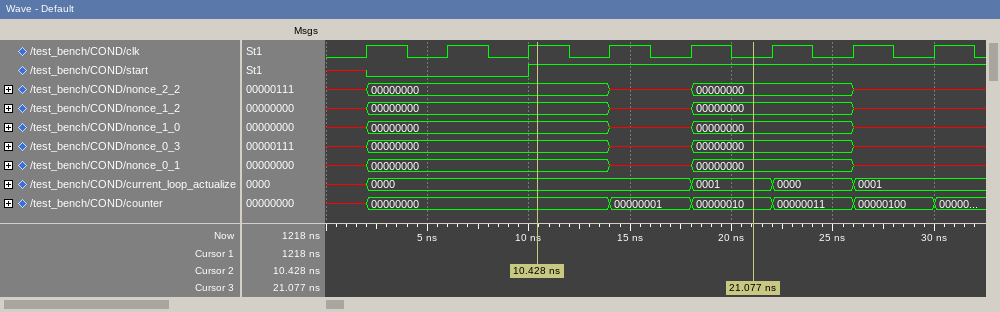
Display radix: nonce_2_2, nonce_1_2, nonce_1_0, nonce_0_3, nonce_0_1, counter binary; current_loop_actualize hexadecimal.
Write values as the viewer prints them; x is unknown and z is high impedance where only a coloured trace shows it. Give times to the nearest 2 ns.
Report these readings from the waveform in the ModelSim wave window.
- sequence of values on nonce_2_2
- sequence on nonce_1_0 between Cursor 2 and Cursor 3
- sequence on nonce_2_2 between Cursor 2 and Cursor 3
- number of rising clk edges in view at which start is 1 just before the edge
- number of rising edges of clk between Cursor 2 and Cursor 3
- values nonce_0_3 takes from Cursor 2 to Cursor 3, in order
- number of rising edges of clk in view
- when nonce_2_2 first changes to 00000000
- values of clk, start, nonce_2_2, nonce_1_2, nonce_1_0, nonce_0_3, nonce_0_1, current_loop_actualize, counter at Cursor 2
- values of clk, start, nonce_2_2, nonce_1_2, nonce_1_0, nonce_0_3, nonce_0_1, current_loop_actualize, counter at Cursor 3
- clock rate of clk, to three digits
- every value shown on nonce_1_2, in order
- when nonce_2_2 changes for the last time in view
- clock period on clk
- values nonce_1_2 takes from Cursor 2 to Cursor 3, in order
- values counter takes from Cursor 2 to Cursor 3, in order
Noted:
x, 00000000, x, 00000000, x
00000000, x, 00000000
00000000, x, 00000000
5
2
00000000, x, 00000000
8
2 ns
clk=1, start=1, nonce_2_2=00000000, nonce_1_2=00000000, nonce_1_0=00000000, nonce_0_3=00000000, nonce_0_1=00000000, current_loop_actualize=0000, counter=00000000
clk=0, start=1, nonce_2_2=00000000, nonce_1_2=00000000, nonce_1_0=00000000, nonce_0_3=00000000, nonce_0_1=00000000, current_loop_actualize=0001, counter=00000010
250 MHz
x, 00000000, x, 00000000, x
26 ns
4 ns
00000000, x, 00000000
00000000, 00000001, 00000010
